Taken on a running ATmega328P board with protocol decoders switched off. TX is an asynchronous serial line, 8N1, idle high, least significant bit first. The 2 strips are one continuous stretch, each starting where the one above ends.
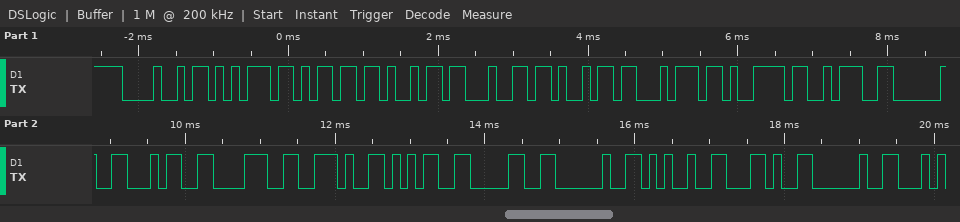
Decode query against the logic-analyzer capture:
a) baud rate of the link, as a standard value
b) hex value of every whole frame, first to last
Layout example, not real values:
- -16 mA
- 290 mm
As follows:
- 9600 baud
- 0x48 0x75 0x6D 0x69 0x64 0x69 0x74 0x79 0x3A 0x20 0x34 0x38 0x2E 0x35 0x30 0x20 0x25 0x2C 0x20
